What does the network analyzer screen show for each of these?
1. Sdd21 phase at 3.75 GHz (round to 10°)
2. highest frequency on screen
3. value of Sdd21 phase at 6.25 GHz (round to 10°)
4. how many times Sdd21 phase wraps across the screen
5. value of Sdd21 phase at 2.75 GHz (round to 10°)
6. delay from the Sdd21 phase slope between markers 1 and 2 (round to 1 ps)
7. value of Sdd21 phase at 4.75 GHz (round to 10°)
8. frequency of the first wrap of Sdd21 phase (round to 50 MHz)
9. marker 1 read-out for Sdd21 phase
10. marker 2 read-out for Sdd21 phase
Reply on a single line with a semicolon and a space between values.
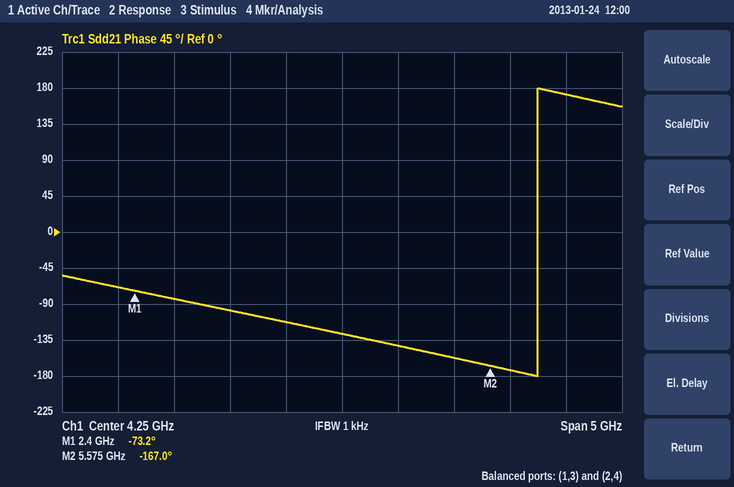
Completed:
-110°; 6.75 GHz; 170°; 1; -80°; 82 ps; -140°; 6.00 GHz; -73.2°; -167.0°
